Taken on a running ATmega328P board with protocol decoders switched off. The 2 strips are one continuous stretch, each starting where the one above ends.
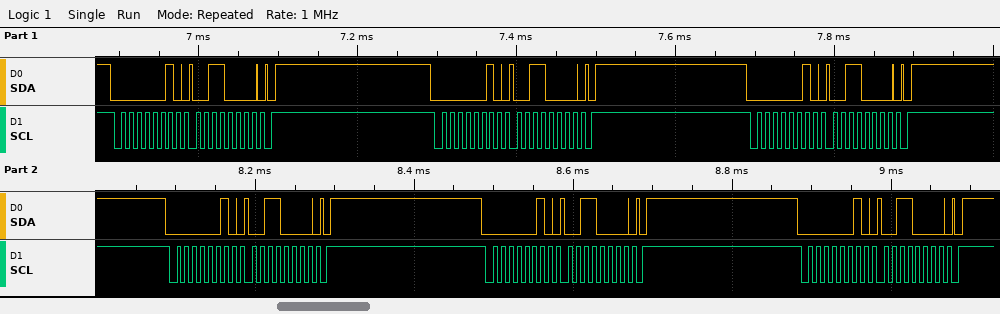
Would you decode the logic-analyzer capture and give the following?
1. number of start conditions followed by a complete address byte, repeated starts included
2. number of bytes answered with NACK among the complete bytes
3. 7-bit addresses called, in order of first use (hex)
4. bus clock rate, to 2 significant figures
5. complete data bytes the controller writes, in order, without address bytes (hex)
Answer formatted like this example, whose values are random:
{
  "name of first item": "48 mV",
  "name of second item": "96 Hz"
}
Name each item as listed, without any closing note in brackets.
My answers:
{
  "number of start conditions followed by a complete address byte, repeated starts included": "6",
  "number of bytes answered with NACK among the complete bytes": "0",
  "7-bit addresses called, in order of first use": "0x01",
  "bus clock rate, to 2 significant figures": "100 kHz",
  "complete data bytes the controller writes, in order, without address bytes": "30 30 30 30 30 30"
}
